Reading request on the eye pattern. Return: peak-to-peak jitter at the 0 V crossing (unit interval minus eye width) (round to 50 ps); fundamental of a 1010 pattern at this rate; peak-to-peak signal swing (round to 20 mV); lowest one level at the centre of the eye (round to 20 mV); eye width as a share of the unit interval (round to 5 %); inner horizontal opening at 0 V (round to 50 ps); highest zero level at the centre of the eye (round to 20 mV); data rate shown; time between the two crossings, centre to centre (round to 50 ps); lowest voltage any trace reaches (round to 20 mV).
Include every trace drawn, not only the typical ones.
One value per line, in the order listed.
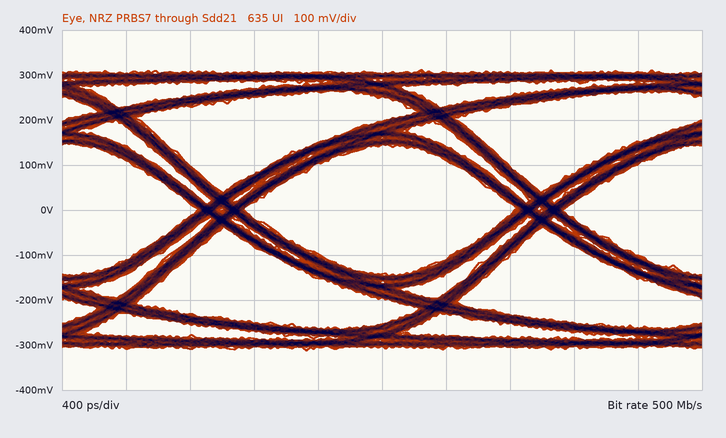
300 ps
250 MHz
620 mV
140 mV
85 %
1.70 ns
-140 mV
500 Mb/s
2.00 ns
-320 mV
